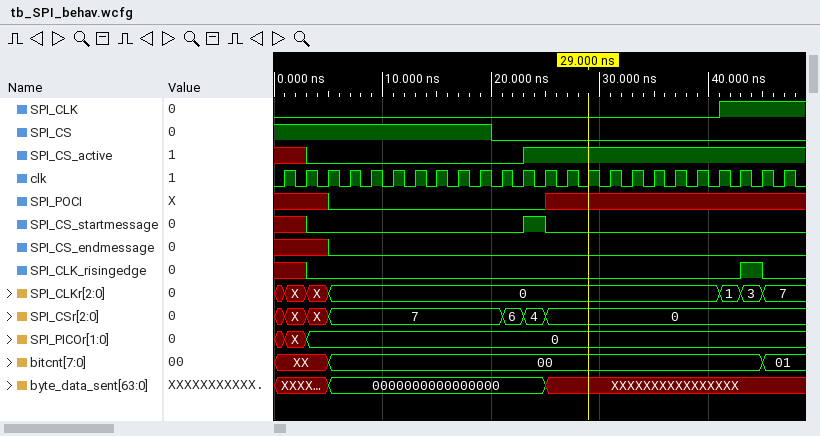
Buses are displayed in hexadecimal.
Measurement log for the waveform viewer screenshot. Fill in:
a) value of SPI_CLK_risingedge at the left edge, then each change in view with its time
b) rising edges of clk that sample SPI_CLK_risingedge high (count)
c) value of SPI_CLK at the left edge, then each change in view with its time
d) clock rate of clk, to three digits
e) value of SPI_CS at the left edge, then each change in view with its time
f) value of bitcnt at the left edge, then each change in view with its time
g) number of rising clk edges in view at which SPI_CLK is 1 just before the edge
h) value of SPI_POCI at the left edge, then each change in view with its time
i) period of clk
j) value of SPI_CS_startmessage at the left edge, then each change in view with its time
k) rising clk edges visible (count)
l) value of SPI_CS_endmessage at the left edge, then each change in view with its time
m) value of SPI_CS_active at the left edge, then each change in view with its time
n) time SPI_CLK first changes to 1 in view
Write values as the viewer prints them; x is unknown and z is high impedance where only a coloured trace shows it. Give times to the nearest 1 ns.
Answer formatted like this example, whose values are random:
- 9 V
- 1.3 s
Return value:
- x, 0 at 3 ns, 1 at 43 ns, 0 at 45 ns
- 1
- 0, 1 at 41 ns
- 500 MHz
- 1, 0 at 20 ns
- XX, 00 at 5 ns, 01 at 45 ns
- 3
- x, 0 at 5 ns, x at 25 ns
- 2 ns
- x, 0 at 3 ns, 1 at 23 ns, 0 at 25 ns
- 24
- x, 0 at 5 ns
- x, 0 at 3 ns, 1 at 23 ns
- 41 ns
